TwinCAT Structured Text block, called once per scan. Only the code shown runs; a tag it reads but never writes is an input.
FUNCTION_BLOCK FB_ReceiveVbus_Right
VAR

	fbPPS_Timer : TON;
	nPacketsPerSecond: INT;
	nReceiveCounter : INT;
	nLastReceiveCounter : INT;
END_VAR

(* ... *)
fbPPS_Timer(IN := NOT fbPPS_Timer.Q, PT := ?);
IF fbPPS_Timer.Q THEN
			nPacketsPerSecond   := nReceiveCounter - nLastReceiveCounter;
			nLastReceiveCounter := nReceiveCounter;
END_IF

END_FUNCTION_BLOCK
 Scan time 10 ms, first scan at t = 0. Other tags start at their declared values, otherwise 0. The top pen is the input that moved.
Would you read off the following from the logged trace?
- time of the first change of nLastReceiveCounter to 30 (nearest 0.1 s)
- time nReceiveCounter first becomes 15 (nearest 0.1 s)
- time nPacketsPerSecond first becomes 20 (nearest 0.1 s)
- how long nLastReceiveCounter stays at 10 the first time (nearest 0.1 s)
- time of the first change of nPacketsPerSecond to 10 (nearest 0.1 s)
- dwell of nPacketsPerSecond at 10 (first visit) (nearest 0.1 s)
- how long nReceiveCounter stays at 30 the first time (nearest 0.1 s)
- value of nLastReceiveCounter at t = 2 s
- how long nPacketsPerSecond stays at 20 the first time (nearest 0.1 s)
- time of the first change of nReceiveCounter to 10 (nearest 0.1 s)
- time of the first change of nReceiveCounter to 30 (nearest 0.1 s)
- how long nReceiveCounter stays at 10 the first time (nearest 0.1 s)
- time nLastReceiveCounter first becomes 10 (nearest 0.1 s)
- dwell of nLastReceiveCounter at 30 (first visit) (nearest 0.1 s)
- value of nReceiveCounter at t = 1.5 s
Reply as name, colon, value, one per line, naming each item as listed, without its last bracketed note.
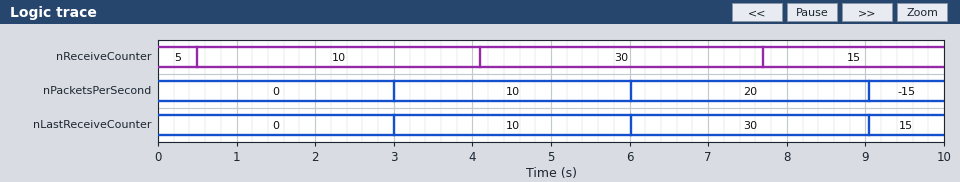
time of the first change of nLastReceiveCounter to 30: 6.0 s
time nReceiveCounter first becomes 15: 7.7 s
time nPacketsPerSecond first becomes 20: 6.0 s
how long nLastReceiveCounter stays at 10 the first time: 3.0 s
time of the first change of nPacketsPerSecond to 10: 3.0 s
dwell of nPacketsPerSecond at 10 (first visit): 3.0 s
how long nReceiveCounter stays at 30 the first time: 3.6 s
value of nLastReceiveCounter at t = 2 s: 0
how long nPacketsPerSecond stays at 20 the first time: 3.0 s
time of the first change of nReceiveCounter to 10: 0.5 s
time of the first change of nReceiveCounter to 30: 4.1 s
how long nReceiveCounter stays at 10 the first time: 3.6 s
time nLastReceiveCounter first becomes 10: 3.0 s
dwell of nLastReceiveCounter at 30 (first visit): 3.0 s
value of nReceiveCounter at t = 1.5 s: 10
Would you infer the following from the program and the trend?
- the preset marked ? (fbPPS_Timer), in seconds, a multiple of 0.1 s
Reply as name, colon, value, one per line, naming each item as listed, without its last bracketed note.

the preset marked ? (fbPPS_Timer), in seconds, a multiple of 0.1 s: 3.0 s
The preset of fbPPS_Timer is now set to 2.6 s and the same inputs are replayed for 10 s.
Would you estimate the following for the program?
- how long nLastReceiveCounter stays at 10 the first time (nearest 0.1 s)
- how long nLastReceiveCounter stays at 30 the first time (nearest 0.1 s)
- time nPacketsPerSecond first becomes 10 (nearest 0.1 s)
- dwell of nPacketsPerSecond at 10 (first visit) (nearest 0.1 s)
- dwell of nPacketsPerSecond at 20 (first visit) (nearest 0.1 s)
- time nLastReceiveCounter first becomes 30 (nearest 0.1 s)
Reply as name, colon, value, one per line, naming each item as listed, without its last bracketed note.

how long nLastReceiveCounter stays at 10 the first time: 2.6 s
how long nLastReceiveCounter stays at 30 the first time: 2.6 s
time nPacketsPerSecond first becomes 10: 2.6 s
dwell of nPacketsPerSecond at 10 (first visit): 2.6 s
dwell of nPacketsPerSecond at 20 (first visit): 2.6 s
time nLastReceiveCounter first becomes 30: 5.2 s
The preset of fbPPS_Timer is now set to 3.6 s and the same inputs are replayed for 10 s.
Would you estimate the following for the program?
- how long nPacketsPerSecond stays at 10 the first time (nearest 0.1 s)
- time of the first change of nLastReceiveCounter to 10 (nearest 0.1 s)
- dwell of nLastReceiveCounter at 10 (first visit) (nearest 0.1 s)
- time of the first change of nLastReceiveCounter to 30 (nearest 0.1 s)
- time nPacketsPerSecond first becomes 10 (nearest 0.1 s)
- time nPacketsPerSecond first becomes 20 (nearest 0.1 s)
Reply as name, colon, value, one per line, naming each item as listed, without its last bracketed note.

how long nPacketsPerSecond stays at 10 the first time: 3.6 s
time of the first change of nLastReceiveCounter to 10: 3.6 s
dwell of nLastReceiveCounter at 10 (first visit): 3.6 s
time of the first change of nLastReceiveCounter to 30: 7.2 s
time nPacketsPerSecond first becomes 10: 3.6 s
time nPacketsPerSecond first becomes 20: 7.2 s
